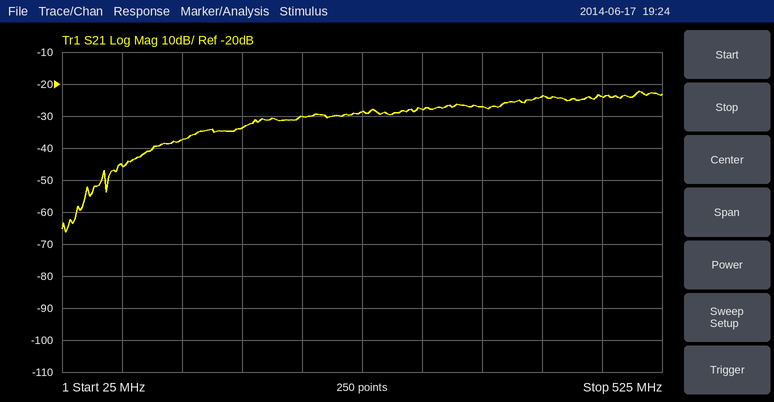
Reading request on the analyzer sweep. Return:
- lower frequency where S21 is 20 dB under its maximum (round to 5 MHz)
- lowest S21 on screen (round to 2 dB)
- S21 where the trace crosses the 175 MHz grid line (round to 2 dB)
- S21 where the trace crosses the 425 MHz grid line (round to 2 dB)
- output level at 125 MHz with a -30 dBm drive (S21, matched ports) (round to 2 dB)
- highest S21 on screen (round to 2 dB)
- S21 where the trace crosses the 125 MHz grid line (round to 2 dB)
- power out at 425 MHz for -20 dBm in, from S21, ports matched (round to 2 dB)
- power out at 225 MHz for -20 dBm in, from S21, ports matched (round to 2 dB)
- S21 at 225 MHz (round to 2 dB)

90 MHz
-66 dB
-34 dB
-24 dB
-68 dBm
-22 dB
-38 dB
-44 dBm
-50 dBm
-30 dB
